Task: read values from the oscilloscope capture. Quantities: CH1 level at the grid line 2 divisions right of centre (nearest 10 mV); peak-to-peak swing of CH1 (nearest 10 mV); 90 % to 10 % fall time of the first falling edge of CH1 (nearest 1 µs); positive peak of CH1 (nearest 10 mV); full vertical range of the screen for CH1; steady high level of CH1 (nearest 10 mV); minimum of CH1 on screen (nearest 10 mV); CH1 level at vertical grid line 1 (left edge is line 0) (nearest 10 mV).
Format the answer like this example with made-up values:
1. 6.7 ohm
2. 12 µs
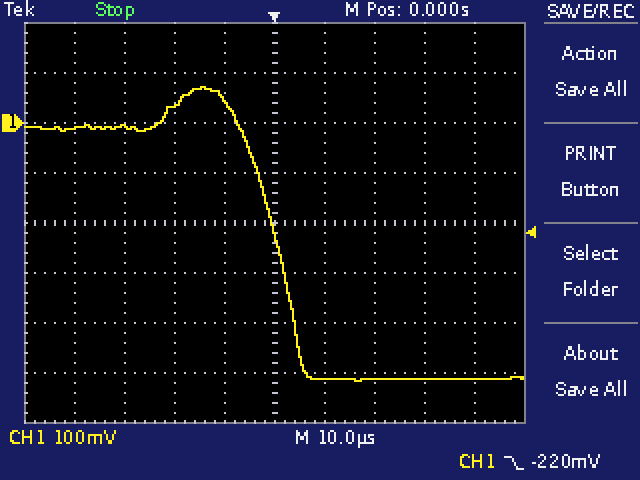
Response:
1. -510 mV
2. 590 mV
3. 10 µs
4. 70 mV
5. 800 mV
6. -10 mV
7. -520 mV
8. -10 mV
